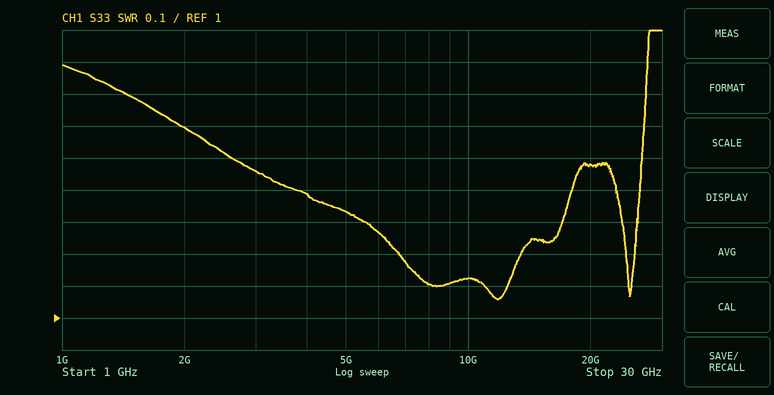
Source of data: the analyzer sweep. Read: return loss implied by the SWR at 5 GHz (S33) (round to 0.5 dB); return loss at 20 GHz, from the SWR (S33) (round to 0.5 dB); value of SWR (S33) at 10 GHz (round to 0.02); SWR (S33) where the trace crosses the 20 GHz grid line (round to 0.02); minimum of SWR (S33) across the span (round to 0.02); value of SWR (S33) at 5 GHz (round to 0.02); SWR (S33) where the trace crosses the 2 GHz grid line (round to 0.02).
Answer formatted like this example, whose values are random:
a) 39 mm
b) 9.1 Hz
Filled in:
a) 17.0 dB
b) 14.5 dB
c) 1.12
d) 1.48
e) 1.06
f) 1.34
g) 1.60
